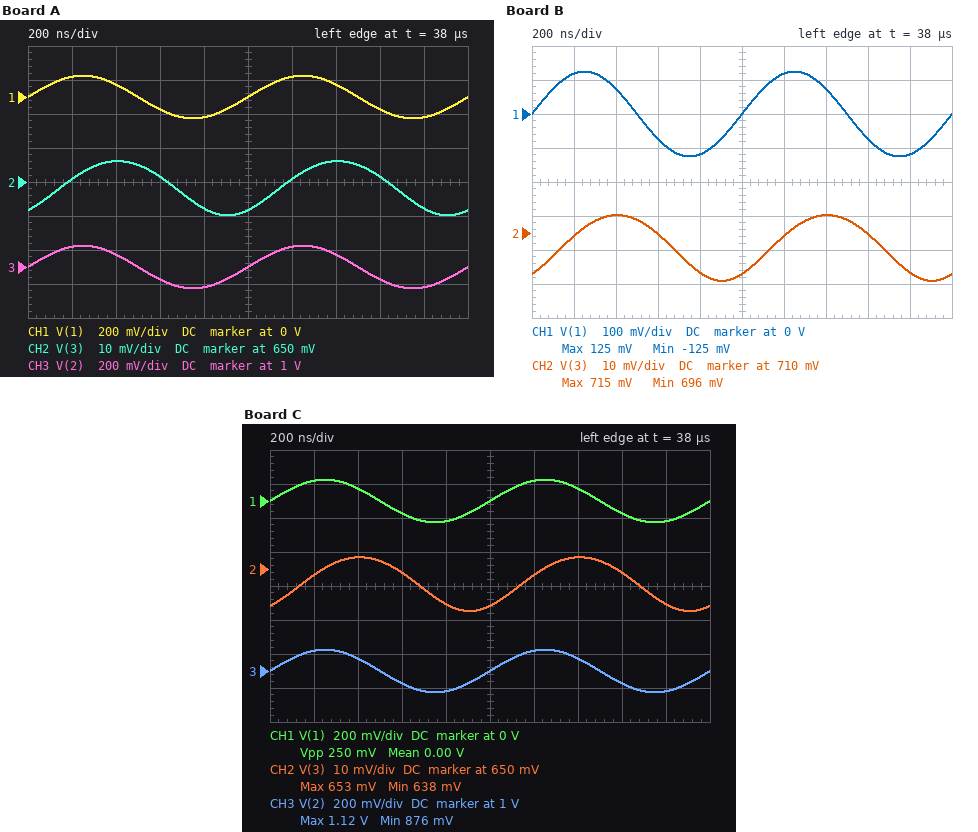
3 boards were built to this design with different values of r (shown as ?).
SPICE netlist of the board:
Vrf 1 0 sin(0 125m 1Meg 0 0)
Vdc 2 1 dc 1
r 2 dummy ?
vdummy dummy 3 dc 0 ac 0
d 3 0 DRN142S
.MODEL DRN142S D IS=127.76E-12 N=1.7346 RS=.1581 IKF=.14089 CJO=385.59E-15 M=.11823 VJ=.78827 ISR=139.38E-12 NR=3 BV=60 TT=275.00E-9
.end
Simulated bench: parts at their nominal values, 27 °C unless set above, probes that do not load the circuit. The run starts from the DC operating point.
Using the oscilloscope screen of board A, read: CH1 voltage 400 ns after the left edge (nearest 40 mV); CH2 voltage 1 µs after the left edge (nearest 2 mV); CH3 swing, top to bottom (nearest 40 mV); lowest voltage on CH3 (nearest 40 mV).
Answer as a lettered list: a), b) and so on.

a) 80 mV
b) 642 mV
c) 240 mV
d) 880 mV
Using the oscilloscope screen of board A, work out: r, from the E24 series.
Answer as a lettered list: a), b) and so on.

a) 1.5 kΩ
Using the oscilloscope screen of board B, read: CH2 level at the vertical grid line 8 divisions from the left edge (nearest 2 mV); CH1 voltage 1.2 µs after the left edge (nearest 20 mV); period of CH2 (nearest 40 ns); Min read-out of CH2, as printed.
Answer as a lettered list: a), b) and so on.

a) 710 mV
b) 120 mV
c) 1.00 µs
d) 696 mV
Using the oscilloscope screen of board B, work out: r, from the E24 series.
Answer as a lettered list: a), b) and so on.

a) 360 Ω
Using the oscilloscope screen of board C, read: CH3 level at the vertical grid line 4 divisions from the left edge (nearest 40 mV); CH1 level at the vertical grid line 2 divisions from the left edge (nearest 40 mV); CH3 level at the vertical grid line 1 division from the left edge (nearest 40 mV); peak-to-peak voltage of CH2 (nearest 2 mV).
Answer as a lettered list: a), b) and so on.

a) 880 mV
b) 80 mV
c) 1.12 V
d) 16 mV
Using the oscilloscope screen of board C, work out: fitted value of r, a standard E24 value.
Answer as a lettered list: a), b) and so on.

a) 1.6 kΩ
